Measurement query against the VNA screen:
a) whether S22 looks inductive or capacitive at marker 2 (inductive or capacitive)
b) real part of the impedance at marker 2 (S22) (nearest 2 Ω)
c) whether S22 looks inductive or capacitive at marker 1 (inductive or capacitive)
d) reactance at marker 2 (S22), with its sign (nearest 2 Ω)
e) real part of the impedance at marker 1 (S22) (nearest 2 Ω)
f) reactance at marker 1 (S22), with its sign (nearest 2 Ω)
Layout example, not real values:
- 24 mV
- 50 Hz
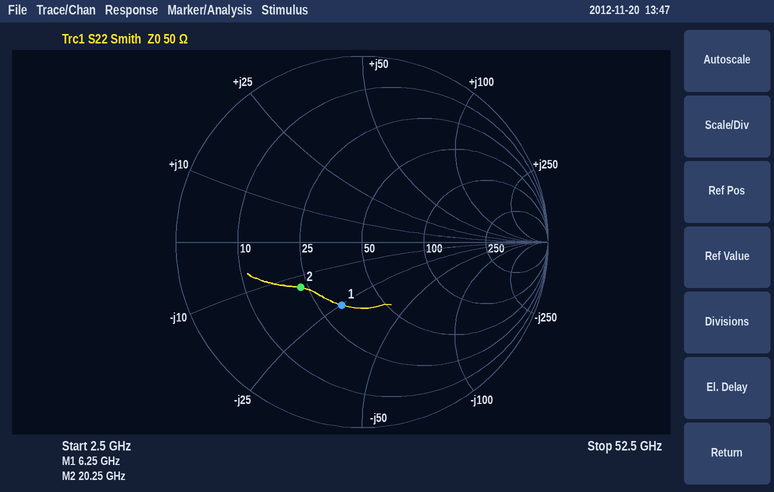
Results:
- capacitive
- 22 Ω
- capacitive
- -14 Ω
- 32 Ω
- -26 Ω
